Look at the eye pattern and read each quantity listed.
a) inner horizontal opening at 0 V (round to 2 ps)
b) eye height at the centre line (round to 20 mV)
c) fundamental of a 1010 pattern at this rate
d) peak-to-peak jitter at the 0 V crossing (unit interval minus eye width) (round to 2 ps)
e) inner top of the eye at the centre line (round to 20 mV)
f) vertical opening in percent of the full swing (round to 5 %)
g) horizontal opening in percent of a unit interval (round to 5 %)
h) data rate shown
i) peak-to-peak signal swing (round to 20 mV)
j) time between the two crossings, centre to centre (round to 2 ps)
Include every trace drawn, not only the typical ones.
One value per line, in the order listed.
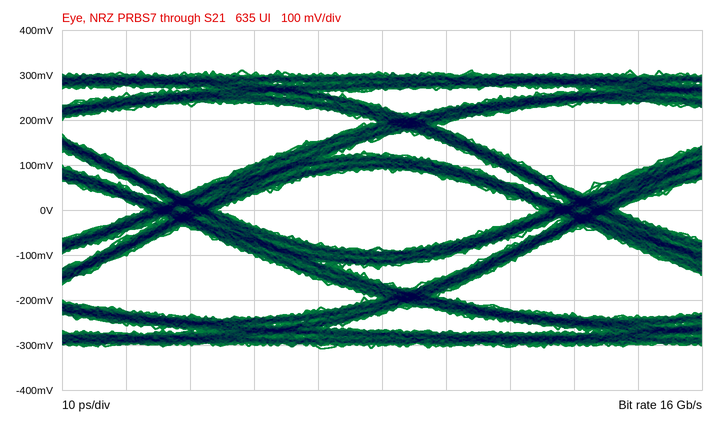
50 ps
180 mV
8 GHz
12 ps
100 mV
30 %
80 %
16 Gb/s
620 mV
62 ps
